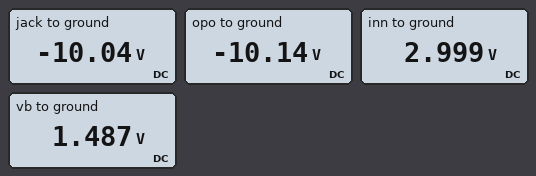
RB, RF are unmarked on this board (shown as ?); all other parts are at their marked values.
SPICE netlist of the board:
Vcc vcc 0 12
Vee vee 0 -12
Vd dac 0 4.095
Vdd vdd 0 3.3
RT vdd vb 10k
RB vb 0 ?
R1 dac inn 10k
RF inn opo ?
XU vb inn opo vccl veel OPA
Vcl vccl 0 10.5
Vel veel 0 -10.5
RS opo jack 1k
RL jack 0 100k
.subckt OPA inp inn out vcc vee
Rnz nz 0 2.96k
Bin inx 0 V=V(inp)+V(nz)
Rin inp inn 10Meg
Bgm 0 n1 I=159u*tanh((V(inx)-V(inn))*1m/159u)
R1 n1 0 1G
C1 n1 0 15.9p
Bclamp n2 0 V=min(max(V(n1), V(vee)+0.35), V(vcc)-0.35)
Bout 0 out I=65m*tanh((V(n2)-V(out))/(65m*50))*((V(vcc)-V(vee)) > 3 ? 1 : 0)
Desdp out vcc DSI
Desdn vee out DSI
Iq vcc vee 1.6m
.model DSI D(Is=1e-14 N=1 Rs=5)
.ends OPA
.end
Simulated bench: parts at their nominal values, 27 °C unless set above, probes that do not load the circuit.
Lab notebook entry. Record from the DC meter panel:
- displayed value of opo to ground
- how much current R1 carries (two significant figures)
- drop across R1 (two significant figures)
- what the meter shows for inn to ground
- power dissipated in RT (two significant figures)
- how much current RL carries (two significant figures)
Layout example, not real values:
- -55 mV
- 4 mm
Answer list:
- -10.14 V
- 110 µA
- 1.1 V
- 2.999 V
- 330 µW
- 100 µA
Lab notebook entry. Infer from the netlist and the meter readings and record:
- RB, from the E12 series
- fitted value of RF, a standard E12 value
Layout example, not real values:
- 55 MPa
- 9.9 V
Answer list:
- 8.2 kΩ
- 120 kΩ
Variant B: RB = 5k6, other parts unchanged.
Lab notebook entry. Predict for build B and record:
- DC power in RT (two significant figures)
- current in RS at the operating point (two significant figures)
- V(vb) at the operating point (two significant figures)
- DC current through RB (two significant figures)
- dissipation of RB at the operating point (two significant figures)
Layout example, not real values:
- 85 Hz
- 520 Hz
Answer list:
- 450 µW
- 100 µA
- 1.2 V
- 210 µA
- 250 µW
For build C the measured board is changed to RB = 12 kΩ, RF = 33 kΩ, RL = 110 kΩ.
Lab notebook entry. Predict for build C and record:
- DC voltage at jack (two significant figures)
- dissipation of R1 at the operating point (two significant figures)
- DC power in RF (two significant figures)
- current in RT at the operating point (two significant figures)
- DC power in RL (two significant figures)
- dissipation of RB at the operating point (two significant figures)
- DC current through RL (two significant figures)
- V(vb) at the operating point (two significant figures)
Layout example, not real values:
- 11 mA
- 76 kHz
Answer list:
- -5.7 V
- 530 µW
- 1.7 mW
- 150 µA
- 300 µW
- 270 µW
- 52 µA
- 1.8 V
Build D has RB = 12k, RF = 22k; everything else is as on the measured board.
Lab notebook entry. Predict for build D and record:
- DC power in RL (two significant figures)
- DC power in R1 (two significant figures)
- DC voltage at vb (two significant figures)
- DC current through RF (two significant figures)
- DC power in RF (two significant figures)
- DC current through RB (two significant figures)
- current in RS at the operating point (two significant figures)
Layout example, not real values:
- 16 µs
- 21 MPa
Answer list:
- 100 µW
- 530 µW
- 1.8 V
- 230 µA
- 1.2 mW
- 150 µA
- 32 µA
